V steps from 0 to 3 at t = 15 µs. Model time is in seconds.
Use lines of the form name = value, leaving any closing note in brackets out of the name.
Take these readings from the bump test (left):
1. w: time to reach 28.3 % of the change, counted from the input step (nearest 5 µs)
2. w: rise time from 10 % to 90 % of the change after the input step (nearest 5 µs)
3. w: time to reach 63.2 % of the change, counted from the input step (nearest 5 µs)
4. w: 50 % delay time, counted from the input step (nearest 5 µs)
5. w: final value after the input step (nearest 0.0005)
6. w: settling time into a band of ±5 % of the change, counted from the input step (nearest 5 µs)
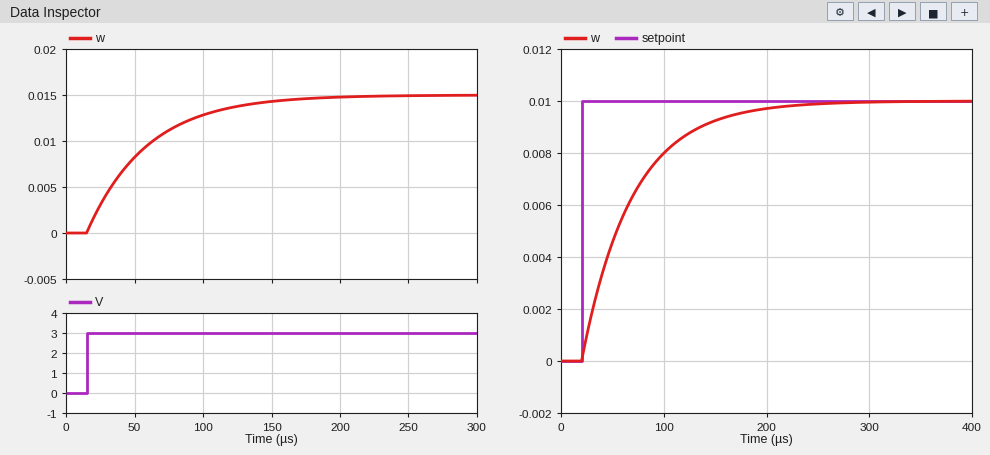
w: time to reach 28.3 % of the change, counted from the input step = 15 µs
w: rise time from 10 % to 90 % of the change after the input step = 95 µs
w: time to reach 63.2 % of the change, counted from the input step = 45 µs
w: 50 % delay time, counted from the input step = 30 µs
w: final value after the input step = 0.0150
w: settling time into a band of ±5 % of the change, counted from the input step = 130 µs
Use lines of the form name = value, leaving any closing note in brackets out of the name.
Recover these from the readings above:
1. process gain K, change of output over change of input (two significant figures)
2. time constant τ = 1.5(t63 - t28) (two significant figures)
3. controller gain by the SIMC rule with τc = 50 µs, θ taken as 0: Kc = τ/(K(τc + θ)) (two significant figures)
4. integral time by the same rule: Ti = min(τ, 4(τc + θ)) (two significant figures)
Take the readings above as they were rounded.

process gain K, change of output over change of input = 0.0050
time constant τ = 1.5(t63 - t28) = 45 µs
controller gain by the SIMC rule with τc = 50 µs, θ taken as 0: Kc = τ/(K(τc + θ)) = 180
integral time by the same rule: Ti = min(τ, 4(τc + θ)) = 45 µs
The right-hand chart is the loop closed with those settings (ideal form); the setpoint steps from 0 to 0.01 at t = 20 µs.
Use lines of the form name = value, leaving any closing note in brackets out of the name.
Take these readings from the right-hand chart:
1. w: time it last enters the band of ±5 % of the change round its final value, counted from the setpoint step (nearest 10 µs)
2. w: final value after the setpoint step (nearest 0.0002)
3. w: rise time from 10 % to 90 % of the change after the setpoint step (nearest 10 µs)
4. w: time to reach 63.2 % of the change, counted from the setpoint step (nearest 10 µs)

w: time it last enters the band of ±5 % of the change round its final value, counted from the setpoint step = 150 µs
w: final value after the setpoint step = 0.0100
w: rise time from 10 % to 90 % of the change after the setpoint step = 110 µs
w: time to reach 63.2 % of the change, counted from the setpoint step = 50 µs
